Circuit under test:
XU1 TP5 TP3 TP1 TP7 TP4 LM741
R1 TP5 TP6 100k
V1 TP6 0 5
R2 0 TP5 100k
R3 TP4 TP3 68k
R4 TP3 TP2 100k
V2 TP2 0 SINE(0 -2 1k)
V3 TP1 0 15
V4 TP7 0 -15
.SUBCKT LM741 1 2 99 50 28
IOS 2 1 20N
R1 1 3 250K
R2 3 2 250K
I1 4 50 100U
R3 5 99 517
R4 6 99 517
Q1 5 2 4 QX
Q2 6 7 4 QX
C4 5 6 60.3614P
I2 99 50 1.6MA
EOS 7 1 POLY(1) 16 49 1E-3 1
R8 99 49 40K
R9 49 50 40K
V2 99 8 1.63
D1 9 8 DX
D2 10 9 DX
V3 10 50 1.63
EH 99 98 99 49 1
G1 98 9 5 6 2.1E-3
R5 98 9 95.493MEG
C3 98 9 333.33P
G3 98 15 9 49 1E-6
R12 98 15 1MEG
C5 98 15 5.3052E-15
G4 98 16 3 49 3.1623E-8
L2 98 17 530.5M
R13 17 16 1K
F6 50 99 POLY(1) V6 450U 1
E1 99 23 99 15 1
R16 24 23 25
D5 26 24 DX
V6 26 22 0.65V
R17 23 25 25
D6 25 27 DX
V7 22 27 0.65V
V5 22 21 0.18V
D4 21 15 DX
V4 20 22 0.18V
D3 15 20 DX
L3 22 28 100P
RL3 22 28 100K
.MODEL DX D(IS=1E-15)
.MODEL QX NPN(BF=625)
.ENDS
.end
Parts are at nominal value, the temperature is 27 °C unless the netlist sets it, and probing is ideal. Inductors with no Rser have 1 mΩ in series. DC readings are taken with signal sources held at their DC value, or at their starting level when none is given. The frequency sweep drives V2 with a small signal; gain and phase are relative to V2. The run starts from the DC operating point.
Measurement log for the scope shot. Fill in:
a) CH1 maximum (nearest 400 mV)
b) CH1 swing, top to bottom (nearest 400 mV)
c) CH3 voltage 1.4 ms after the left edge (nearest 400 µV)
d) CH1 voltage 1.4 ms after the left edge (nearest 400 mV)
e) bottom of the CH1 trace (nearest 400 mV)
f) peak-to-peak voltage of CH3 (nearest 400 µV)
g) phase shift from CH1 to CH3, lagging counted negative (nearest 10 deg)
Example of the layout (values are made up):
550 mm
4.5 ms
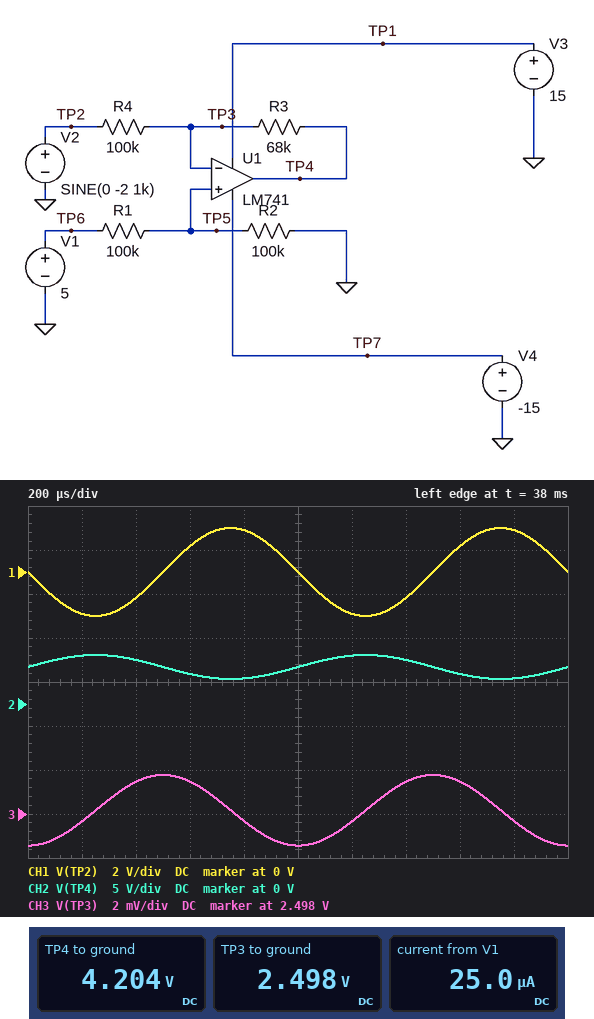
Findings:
2.0 V
4.0 V
2.4996 V
-1.2 V
-2.0 V
3.2 mV
90 deg
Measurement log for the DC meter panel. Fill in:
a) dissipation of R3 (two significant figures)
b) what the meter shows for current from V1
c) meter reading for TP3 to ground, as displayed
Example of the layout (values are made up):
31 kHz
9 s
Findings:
43 µW
25.0 µA
2.498 V
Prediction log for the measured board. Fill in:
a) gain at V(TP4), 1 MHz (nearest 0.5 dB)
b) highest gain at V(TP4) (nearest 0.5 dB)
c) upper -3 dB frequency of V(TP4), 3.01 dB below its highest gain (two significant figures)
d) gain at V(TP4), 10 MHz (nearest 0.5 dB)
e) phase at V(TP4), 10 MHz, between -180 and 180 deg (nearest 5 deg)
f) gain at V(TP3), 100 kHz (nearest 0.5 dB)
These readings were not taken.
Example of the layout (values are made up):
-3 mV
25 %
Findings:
-10.0 dB
-3.5 dB
580 kHz
-40.5 dB
-35 deg
-22.0 dB
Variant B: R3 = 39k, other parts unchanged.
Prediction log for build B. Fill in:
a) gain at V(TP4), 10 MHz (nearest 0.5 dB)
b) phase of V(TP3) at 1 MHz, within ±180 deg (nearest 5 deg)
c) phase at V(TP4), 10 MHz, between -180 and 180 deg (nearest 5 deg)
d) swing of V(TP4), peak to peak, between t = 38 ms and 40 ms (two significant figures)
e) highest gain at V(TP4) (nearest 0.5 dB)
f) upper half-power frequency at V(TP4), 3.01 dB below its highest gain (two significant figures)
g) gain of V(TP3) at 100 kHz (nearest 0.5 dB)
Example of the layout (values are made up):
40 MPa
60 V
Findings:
-43.0 dB
30 deg
-30 deg
1.6 V
-8.0 dB
770 kHz
-27.0 dB
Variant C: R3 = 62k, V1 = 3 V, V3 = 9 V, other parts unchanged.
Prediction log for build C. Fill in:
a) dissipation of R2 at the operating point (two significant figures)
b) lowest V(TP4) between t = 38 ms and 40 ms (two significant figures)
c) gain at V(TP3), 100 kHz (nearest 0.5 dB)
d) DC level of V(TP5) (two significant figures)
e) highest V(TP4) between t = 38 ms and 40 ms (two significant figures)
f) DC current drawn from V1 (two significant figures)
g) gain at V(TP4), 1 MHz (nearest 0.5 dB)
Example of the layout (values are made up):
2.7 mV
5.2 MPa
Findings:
22 µW
1.2 V
-23.0 dB
1.5 V
3.7 V
15 µA
-10.5 dB
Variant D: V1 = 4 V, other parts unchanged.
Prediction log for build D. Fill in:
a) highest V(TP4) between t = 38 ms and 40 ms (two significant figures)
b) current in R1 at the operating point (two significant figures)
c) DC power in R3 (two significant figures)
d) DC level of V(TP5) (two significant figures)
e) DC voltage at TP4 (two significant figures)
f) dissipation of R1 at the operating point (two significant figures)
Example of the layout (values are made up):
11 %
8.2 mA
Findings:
4.7 V
20 µA
27 µW
2.0 V
3.4 V
40 µW
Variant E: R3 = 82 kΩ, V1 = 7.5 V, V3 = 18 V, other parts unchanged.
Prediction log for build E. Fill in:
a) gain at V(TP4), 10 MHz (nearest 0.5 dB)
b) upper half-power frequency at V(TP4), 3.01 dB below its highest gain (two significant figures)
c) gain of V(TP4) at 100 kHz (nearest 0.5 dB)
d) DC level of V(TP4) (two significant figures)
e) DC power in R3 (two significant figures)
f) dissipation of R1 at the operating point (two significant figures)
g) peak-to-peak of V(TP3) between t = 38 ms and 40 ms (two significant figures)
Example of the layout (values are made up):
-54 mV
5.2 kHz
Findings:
-40.0 dB
510 kHz
-2.0 dB
6.8 V
120 µW
140 µW
3.9 mV
